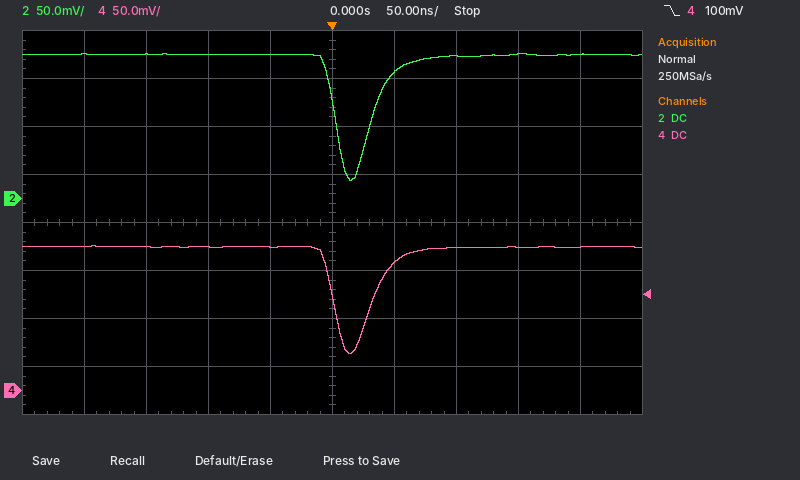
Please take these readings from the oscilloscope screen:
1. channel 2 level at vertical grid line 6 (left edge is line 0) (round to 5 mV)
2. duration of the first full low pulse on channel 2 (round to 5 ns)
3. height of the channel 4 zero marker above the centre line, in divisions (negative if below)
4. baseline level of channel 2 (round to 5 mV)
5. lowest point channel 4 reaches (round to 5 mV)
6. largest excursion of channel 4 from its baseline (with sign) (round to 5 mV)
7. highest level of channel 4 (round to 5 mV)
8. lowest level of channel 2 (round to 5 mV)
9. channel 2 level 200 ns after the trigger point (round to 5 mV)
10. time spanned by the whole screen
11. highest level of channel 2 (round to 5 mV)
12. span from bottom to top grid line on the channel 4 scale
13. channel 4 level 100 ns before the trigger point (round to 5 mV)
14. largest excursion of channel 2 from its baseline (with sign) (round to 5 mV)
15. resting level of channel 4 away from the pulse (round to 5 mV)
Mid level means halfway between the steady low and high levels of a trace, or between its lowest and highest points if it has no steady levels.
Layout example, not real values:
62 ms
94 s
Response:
130 mV
30 ns
-3.5 div
150 mV
40 mV
-110 mV
150 mV
20 mV
150 mV
500 ns
150 mV
400 mV
150 mV
-130 mV
150 mV
